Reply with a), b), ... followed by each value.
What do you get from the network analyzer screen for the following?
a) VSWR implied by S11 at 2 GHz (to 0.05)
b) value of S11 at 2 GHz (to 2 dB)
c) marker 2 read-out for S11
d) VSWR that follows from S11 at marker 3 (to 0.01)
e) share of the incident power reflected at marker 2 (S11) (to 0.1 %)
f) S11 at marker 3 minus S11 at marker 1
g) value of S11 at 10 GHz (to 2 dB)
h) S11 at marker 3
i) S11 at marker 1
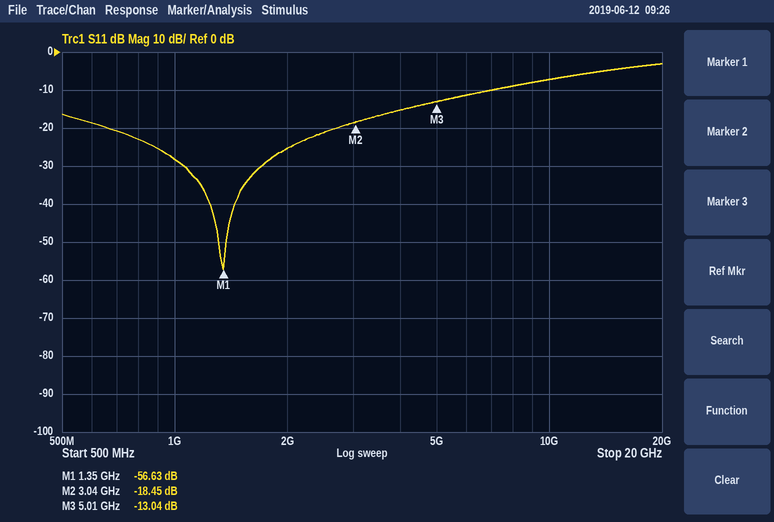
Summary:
a) 1.10
b) -26 dB
c) -18.45 dB
d) 1.57
e) 1.4 %
f) 43.59 dB
g) -8 dB
h) -13.04 dB
i) -56.63 dB
